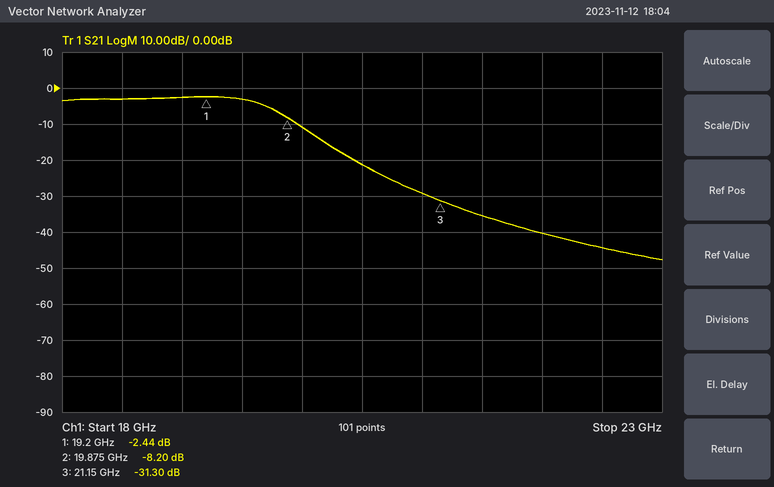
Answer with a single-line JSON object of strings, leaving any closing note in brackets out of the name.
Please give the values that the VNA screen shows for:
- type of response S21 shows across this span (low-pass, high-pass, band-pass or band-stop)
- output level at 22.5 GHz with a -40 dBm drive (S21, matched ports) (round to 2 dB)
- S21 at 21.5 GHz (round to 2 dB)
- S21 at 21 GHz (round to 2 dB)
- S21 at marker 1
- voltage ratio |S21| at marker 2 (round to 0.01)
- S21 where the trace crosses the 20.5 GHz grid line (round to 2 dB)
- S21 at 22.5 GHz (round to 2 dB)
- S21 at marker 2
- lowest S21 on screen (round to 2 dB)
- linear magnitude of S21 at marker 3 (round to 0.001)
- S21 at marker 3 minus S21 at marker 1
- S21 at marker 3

{"type of response S21 shows across this span": "low-pass", "output level at 22.5 GHz with a -40 dBm drive (S21, matched ports)": "-84 dBm", "S21 at 21.5 GHz": "-36 dB", "S21 at 21 GHz": "-30 dB", "S21 at marker 1": "-2.44 dB", "voltage ratio |S21| at marker 2": "0.39", "S21 where the trace crosses the 20.5 GHz grid line": "-22 dB", "S21 at 22.5 GHz": "-44 dB", "S21 at marker 2": "-8.20 dB", "lowest S21 on screen": "-48 dB", "linear magnitude of S21 at marker 3": "0.027", "S21 at marker 3 minus S21 at marker 1": "-28.86 dB", "S21 at marker 3": "-31.30 dB"}
